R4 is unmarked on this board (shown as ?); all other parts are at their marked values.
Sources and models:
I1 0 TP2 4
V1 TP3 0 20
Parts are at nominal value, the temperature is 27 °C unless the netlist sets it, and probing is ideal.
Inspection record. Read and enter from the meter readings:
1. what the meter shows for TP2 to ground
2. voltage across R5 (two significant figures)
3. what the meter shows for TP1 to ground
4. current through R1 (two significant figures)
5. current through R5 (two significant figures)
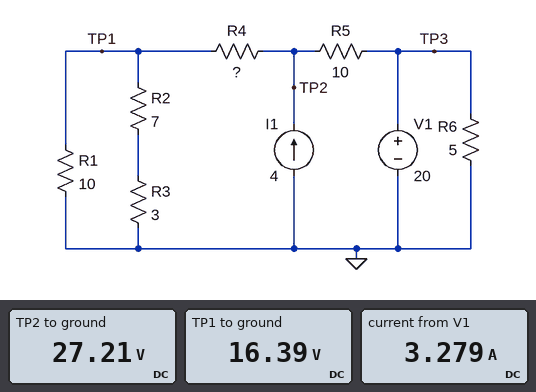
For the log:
27.21 V
7.2 V
16.39 V
1.6 A
720 mA
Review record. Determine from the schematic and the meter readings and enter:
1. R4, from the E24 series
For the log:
3.3 Ω
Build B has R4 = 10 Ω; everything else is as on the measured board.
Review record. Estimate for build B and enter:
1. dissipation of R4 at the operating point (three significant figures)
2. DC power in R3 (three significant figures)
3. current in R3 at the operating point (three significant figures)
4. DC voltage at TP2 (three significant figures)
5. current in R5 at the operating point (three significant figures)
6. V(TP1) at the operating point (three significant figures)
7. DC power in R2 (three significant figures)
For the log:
57.6 W
4.32 W
1.20 A
36.0 V
1.60 A
12.0 V
10.1 W
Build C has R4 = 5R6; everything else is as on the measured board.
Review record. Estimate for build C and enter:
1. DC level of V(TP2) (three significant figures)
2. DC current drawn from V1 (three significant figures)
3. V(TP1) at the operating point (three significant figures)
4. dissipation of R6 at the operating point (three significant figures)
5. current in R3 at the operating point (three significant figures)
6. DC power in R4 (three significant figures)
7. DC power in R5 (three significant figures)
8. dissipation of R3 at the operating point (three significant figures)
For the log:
30.9 V
2.91 A
14.6 V
80.0 W
1.46 A
47.5 W
11.8 W
6.36 W
